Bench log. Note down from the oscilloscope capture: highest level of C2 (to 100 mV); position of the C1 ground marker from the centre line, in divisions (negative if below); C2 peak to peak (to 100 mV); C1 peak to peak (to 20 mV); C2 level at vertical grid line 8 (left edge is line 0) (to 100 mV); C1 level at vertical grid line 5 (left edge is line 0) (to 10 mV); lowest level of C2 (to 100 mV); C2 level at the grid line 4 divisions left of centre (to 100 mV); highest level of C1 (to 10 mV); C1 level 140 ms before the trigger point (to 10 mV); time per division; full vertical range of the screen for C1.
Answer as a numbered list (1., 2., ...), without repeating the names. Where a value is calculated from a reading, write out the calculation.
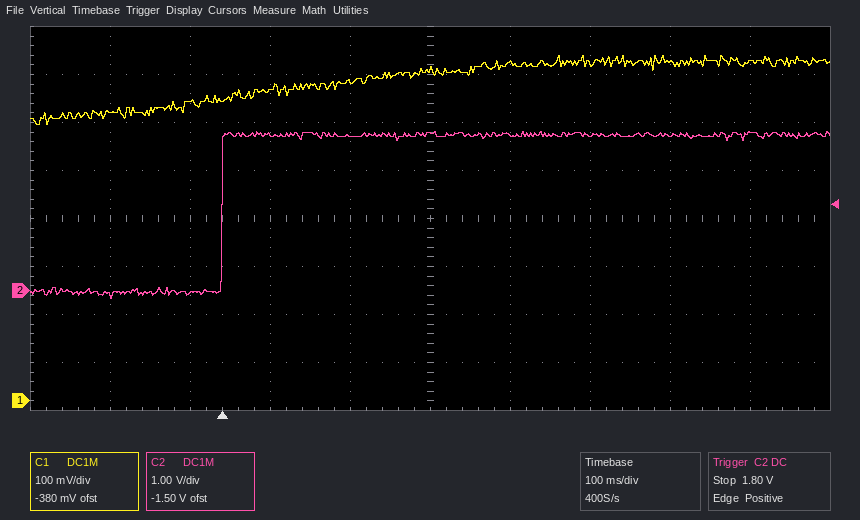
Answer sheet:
1. 3.3 V
2. -3.8 div
3. 3.3 V − (-200 mV) = 3.5 V
4. 140 mV
5. 3.2 V
6. 690 mV
7. -200 mV
8. -100 mV
9. 720 mV
10. 600 mV
11. 100 ms
12. 800 mV
